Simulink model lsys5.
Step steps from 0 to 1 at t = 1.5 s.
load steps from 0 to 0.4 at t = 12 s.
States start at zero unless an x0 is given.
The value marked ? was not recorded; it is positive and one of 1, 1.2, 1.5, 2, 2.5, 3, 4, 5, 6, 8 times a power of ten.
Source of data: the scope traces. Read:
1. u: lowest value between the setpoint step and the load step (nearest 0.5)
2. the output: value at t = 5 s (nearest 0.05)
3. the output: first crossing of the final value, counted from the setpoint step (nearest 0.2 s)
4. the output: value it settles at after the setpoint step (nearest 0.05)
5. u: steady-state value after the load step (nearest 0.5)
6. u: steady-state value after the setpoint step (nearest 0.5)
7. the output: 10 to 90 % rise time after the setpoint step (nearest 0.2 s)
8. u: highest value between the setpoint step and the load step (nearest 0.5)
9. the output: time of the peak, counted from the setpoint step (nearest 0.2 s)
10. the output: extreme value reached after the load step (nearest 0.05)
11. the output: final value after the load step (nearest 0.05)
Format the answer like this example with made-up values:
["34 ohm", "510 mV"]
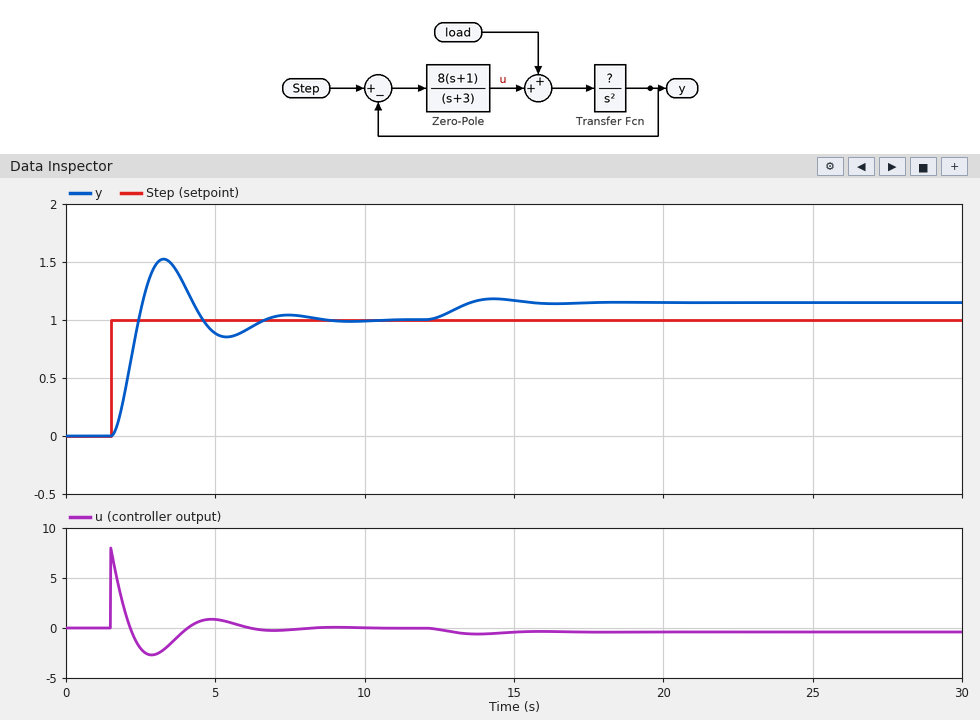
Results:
["-2.5", "0.90", "1.0 s", "1.00", "-0.5", "0.0", "0.6 s", "8.0", "1.8 s", "1.20", "1.15"]
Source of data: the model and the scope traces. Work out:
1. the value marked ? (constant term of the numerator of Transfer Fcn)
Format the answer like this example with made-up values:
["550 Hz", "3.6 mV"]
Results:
["0.6"]
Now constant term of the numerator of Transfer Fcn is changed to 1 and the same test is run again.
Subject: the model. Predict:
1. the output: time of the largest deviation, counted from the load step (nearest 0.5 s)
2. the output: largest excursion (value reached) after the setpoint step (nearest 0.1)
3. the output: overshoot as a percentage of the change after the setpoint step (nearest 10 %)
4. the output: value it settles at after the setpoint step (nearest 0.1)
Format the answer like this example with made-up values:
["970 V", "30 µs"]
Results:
["1.5 s", "1.5", "50 %", "1.0"]
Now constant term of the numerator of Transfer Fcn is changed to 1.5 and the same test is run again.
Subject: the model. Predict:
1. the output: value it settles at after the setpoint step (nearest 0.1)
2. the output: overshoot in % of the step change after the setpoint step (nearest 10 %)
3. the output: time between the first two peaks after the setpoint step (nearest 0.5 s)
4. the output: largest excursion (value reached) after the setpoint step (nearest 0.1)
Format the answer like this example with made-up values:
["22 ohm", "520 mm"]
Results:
["1.0", "60 %", "2.0 s", "1.6"]
